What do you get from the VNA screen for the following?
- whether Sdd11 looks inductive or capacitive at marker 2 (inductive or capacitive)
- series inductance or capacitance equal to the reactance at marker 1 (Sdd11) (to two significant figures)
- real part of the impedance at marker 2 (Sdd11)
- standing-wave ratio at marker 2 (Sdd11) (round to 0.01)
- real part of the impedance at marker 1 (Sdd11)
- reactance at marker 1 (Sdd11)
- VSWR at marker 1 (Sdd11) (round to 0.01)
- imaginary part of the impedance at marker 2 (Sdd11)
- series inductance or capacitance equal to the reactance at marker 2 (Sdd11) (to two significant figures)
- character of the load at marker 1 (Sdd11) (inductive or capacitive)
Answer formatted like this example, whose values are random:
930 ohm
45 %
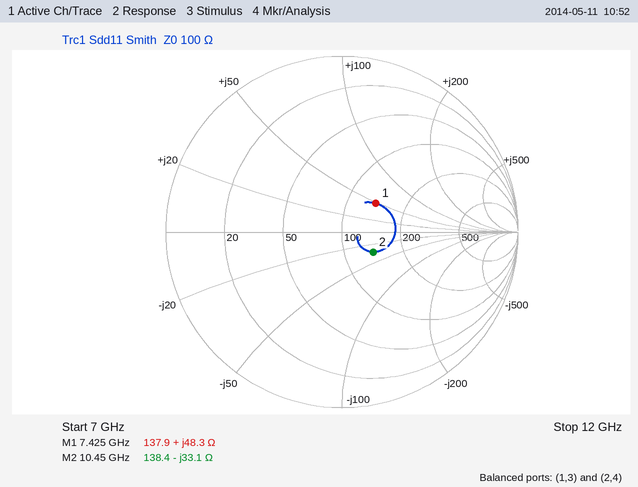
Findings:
capacitive
1.0 nH
138.4 Ω
1.53
137.9 Ω
+48.3 Ω
1.68
-33.1 Ω
460 fF
inductive
